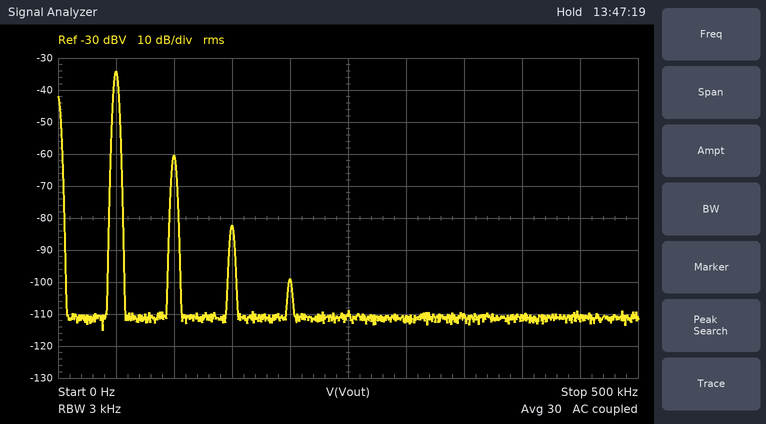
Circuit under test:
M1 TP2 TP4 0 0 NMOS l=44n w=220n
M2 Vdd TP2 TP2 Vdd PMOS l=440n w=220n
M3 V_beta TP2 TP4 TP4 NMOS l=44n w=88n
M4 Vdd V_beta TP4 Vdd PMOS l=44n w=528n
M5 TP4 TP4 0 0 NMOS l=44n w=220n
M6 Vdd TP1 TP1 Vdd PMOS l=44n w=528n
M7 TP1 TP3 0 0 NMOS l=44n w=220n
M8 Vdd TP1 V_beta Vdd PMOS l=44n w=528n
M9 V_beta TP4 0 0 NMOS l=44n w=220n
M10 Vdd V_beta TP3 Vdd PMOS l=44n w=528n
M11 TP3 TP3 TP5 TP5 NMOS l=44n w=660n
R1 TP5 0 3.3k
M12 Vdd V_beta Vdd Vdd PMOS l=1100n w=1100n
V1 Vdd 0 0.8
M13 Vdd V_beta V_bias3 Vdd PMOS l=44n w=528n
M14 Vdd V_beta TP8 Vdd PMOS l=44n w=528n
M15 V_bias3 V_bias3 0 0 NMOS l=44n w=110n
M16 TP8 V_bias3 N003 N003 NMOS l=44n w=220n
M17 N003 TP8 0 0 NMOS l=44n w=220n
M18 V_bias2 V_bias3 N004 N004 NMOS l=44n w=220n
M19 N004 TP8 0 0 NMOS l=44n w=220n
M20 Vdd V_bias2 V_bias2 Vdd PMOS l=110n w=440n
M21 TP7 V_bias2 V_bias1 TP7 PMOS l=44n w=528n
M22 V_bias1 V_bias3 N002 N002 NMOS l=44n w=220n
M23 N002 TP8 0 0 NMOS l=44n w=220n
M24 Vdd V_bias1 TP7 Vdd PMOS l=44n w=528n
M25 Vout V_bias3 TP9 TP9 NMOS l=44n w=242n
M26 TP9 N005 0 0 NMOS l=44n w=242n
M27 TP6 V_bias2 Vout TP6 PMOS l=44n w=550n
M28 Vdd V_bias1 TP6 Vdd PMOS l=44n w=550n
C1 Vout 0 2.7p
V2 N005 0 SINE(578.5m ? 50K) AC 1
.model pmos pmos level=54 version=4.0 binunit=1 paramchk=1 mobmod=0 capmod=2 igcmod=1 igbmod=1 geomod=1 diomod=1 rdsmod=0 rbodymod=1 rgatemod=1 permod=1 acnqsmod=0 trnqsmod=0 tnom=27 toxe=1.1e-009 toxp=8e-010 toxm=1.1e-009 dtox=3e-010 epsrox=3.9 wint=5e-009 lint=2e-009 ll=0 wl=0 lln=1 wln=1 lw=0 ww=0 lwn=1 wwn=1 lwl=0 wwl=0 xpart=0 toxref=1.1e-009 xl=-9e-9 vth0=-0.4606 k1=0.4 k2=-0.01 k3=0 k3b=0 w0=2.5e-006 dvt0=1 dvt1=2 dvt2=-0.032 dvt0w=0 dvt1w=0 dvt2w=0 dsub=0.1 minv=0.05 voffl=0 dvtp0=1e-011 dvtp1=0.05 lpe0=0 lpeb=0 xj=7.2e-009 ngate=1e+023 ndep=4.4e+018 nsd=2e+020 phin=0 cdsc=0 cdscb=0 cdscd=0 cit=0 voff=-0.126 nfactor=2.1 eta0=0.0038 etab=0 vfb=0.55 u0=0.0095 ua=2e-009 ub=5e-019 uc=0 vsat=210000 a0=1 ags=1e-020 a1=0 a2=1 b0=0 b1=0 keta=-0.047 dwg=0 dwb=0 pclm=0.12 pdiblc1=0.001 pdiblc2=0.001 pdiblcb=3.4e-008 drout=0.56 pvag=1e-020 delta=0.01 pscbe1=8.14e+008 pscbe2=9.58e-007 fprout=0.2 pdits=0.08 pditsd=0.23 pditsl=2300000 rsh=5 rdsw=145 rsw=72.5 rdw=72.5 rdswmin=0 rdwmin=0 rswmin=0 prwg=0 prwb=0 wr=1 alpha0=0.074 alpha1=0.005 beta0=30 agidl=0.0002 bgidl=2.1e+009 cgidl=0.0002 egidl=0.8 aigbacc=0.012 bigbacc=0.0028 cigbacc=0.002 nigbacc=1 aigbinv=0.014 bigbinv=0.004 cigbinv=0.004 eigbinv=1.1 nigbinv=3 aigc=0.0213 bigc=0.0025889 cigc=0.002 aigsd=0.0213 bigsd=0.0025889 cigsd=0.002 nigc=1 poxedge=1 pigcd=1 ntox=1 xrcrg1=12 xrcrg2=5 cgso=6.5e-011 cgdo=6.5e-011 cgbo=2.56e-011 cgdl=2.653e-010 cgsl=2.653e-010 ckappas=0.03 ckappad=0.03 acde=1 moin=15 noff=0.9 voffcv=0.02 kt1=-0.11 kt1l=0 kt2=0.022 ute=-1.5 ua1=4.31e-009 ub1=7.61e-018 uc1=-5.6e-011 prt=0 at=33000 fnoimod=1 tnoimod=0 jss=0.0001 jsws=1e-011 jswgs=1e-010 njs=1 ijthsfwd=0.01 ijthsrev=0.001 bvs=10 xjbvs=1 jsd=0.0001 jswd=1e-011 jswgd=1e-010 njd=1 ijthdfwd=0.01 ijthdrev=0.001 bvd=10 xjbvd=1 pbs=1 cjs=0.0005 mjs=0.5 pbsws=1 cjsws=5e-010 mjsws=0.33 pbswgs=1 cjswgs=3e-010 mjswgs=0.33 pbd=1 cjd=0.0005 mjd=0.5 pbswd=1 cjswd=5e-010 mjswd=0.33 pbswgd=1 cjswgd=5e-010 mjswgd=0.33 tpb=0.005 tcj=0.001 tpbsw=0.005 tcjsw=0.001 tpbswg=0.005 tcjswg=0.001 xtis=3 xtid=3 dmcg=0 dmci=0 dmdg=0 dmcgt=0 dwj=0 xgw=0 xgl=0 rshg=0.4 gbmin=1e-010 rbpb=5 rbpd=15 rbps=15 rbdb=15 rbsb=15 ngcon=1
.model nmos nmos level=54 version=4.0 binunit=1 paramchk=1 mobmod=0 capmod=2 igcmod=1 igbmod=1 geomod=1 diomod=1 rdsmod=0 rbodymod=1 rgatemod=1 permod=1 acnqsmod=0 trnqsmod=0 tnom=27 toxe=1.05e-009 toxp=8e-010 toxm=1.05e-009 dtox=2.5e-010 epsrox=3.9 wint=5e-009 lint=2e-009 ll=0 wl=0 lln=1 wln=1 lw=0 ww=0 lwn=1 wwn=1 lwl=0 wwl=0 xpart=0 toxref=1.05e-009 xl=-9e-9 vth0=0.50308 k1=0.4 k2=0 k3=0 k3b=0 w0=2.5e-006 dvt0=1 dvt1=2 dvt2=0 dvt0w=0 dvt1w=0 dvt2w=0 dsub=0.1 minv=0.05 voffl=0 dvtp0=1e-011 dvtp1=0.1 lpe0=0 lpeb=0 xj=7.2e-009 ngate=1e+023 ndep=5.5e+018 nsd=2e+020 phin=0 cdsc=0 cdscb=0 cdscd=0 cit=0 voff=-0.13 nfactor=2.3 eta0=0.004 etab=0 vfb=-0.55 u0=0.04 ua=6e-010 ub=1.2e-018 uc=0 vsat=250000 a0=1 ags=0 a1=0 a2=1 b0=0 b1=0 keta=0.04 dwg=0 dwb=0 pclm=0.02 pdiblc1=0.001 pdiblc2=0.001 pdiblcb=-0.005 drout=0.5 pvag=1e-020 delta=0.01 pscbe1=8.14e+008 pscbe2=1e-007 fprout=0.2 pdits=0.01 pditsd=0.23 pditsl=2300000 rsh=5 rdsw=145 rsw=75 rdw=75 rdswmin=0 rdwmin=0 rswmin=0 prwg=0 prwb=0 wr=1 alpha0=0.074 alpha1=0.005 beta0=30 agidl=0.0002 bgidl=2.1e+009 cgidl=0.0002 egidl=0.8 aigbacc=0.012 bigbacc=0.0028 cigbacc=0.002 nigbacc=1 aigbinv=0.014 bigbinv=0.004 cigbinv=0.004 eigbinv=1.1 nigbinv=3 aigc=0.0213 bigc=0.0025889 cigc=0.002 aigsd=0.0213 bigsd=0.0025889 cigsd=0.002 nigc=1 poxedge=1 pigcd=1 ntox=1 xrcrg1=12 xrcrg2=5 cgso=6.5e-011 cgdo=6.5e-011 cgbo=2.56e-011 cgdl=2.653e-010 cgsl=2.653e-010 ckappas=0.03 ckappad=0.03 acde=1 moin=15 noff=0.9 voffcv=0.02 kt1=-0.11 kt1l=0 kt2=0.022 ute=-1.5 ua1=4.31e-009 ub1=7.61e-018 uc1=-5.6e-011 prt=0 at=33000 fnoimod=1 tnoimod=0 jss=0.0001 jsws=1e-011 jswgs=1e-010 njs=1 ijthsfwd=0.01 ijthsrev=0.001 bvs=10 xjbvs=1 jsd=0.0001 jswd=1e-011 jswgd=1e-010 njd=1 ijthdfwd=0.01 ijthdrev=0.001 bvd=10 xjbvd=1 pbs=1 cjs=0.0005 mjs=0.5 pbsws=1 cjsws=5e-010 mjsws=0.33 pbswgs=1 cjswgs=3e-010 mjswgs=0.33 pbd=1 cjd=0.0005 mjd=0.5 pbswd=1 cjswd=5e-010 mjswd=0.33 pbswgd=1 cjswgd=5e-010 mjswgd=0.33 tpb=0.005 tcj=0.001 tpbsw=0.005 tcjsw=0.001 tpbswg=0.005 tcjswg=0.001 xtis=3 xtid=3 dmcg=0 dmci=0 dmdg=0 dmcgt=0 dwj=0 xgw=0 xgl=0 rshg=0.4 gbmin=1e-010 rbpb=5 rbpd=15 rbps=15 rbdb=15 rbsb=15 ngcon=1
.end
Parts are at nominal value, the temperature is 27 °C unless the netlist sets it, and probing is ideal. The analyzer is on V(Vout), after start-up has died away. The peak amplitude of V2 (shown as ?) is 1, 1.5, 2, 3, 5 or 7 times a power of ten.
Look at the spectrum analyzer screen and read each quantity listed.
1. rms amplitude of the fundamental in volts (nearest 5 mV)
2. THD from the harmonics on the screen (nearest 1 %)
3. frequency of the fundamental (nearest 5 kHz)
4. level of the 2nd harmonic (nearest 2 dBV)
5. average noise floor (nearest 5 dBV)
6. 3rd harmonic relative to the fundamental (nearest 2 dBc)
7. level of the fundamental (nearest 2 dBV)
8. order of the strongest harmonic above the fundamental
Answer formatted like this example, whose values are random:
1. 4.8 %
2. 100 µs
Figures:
1. 20 mV
2. 5 %
3. 50 kHz
4. -60 dBV
5. -110 dBV
6. -48 dBc
7. -34 dBV
8. 2
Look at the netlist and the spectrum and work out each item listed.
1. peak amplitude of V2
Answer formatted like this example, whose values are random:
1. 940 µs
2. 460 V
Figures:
1. 10 mV
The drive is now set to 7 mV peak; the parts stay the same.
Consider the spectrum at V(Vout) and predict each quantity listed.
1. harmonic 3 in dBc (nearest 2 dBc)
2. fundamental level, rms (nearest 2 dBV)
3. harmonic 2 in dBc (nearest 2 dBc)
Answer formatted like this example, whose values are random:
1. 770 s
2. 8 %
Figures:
1. -54 dBc
2. -38 dBV
3. -30 dBc
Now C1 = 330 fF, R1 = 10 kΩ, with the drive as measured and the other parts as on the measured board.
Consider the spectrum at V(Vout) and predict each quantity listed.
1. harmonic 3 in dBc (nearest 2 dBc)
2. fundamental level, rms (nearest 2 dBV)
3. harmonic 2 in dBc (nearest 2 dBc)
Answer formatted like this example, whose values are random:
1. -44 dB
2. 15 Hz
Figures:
1. -42 dBc
2. -46 dBV
3. -22 dBc
